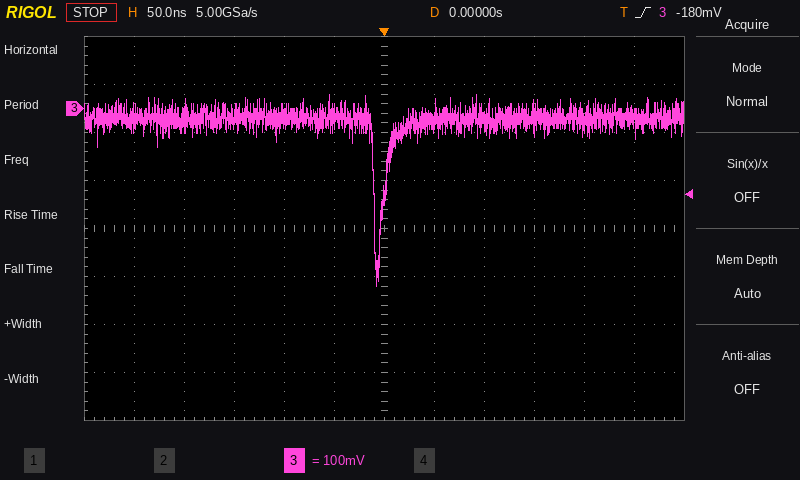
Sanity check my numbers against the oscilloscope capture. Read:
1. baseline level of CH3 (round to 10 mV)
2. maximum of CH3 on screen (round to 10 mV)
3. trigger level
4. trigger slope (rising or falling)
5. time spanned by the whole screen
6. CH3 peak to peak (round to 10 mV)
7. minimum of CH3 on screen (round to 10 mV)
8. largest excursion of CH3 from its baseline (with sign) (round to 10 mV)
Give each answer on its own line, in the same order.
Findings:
-20 mV
30 mV
-180 mV
rising
600 ns
400 mV
-370 mV
-350 mV
